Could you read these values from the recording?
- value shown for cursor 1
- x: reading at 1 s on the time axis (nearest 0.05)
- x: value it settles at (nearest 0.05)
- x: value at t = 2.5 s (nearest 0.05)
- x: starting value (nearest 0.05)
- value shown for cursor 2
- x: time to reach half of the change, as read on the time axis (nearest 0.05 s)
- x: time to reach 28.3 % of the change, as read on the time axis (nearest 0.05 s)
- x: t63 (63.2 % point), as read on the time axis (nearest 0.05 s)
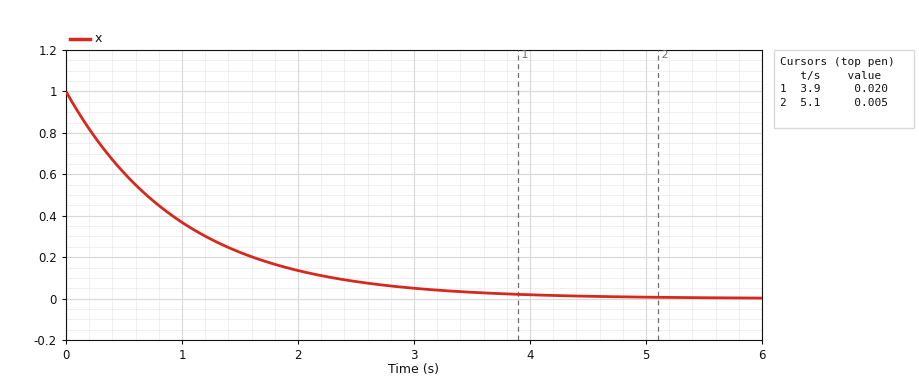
0.020
0.35
0.00
0.10
1.00
0.005
0.70 s
0.35 s
1.00 s
